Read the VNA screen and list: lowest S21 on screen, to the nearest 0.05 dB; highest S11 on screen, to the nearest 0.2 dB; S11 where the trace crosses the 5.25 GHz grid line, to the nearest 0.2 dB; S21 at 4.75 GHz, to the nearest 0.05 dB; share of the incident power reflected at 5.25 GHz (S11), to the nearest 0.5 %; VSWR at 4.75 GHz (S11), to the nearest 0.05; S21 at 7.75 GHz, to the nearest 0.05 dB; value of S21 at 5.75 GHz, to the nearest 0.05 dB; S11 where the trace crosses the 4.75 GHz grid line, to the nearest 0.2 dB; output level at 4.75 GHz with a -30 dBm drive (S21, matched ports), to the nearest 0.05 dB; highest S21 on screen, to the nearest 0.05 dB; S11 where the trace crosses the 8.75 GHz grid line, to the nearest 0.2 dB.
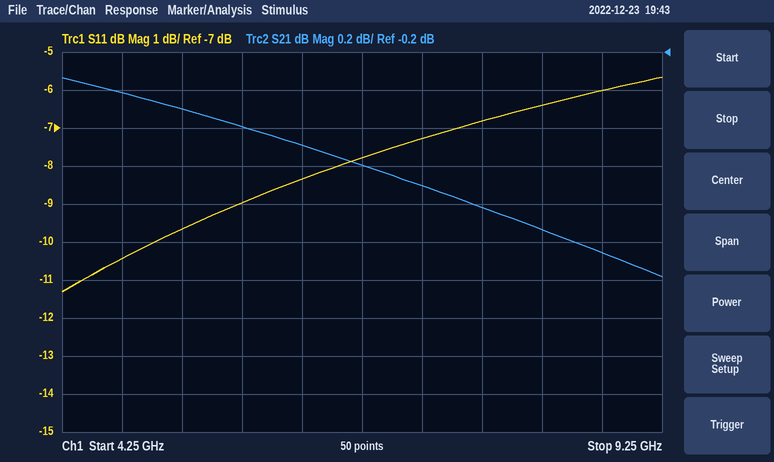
-1.40 dB
-5.6 dB
-9.6 dB
-0.40 dB
11.0 %
1.85
-1.00 dB
-0.60 dB
-10.4 dB
-30.40 dBm
-0.35 dB
-6.0 dB
